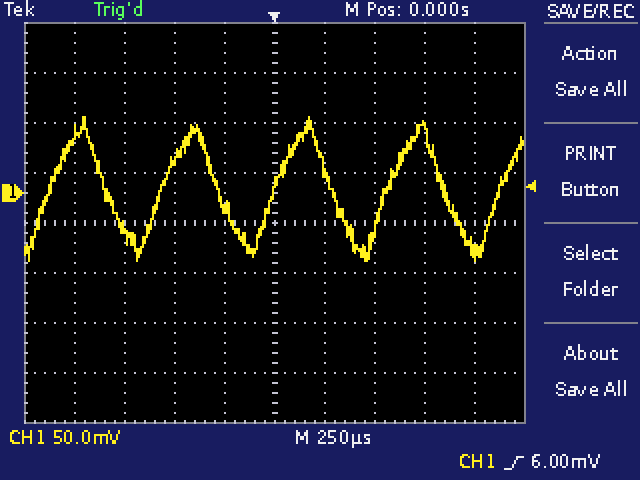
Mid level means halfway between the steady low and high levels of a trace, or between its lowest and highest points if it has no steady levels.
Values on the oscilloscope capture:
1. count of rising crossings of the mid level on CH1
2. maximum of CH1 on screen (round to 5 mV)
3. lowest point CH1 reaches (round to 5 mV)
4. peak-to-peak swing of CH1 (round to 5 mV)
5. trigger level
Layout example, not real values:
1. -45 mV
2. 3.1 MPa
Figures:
1. 5
2. 75 mV
3. -70 mV
4. 145 mV
5. 6.00 mV
